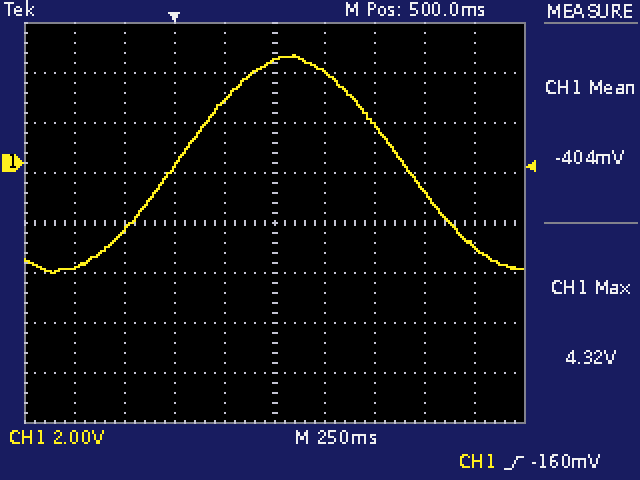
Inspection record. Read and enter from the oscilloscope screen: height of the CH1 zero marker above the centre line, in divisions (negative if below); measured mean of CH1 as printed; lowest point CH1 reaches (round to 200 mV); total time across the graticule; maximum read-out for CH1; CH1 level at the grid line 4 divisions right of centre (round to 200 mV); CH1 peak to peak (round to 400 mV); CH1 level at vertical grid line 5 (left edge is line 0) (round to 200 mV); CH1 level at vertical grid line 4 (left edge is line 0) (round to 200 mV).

+1.2 div
-404 mV
-4.4 V
2.5 s
4.32 V
-3.4 V
8.8 V
4.0 V
2.4 V
